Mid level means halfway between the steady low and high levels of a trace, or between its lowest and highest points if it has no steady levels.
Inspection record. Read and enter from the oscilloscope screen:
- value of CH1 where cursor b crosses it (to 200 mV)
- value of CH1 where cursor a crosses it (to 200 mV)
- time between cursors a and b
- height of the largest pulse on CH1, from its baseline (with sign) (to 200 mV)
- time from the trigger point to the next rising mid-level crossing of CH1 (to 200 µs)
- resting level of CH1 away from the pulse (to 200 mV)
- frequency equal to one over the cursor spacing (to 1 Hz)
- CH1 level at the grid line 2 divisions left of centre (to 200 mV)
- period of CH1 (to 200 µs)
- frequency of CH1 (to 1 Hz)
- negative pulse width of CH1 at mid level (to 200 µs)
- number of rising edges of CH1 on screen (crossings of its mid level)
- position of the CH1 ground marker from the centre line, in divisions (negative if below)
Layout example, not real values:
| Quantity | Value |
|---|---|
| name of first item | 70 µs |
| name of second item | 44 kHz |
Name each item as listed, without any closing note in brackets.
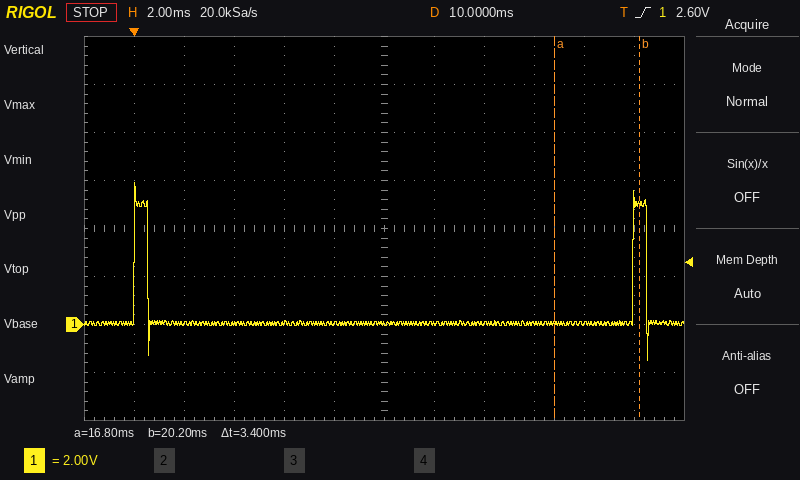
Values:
| Quantity | Value |
|---|---|
| value of CH1 where cursor b crosses it | 5.0 V |
| value of CH1 where cursor a crosses it | 0.0 V |
| time between cursors a and b | 3.4 ms |
| height of the largest pulse on CH1, from its baseline (with sign) | +5.8 V |
| time from the trigger point to the next rising mid-level crossing of CH1 | 20.0 ms |
| resting level of CH1 away from the pulse | 0.0 V |
| frequency equal to one over the cursor spacing | 294 Hz |
| CH1 level at the grid line 2 divisions left of centre | 0.0 V |
| period of CH1 | 20.0 ms |
| frequency of CH1 | 50 Hz |
| negative pulse width of CH1 at mid level | 19.4 ms |
| number of rising edges of CH1 on screen | 2 |
| position of the CH1 ground marker from the centre line, in divisions | -2.0 div |
